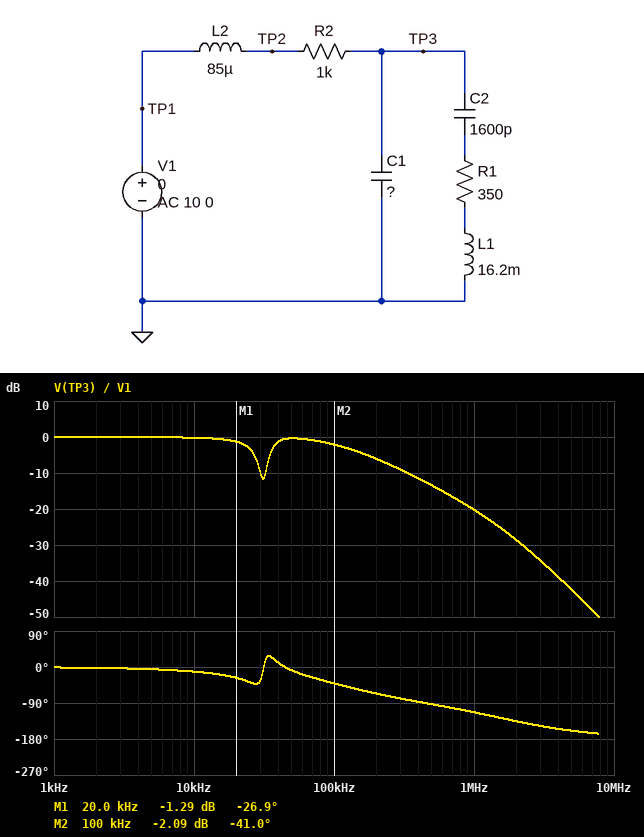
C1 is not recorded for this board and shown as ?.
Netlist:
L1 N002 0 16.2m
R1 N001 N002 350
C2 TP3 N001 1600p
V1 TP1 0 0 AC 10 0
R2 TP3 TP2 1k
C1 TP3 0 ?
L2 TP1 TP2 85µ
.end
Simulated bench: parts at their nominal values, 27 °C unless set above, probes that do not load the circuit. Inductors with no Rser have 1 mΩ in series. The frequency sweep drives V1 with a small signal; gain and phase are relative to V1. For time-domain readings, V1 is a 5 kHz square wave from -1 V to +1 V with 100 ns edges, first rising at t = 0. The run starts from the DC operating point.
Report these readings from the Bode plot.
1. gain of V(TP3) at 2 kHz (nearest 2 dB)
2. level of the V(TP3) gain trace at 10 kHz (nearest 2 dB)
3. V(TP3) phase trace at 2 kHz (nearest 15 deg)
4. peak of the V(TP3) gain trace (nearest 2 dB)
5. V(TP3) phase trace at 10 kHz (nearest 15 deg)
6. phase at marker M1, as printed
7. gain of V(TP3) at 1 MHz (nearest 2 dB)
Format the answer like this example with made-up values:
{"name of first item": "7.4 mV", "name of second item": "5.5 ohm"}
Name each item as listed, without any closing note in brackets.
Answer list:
{"gain of V(TP3) at 2 kHz": "0 dB", "level of the V(TP3) gain trace at 10 kHz": "0 dB", "V(TP3) phase trace at 2 kHz": "0 deg", "peak of the V(TP3) gain trace": "0 dB", "V(TP3) phase trace at 10 kHz": "-15 deg", "phase at marker M1, as printed": "-26.9 deg", "gain of V(TP3) at 1 MHz": "-20 dB"}
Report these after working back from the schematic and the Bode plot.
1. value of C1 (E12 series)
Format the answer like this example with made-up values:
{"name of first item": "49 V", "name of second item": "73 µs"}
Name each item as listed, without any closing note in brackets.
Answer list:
{"value of C1": "1.5 nF"}
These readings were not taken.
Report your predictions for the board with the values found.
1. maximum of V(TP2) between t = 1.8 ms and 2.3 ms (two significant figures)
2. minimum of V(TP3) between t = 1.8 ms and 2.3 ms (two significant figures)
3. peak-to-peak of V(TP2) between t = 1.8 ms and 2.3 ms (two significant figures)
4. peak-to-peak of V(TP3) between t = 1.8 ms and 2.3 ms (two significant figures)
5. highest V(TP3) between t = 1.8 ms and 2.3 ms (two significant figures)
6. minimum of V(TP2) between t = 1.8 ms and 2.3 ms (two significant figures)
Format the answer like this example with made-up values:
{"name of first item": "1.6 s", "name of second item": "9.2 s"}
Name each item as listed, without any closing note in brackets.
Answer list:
{"maximum of V(TP2) between t = 1.8 ms and 2.3 ms": "1.1 V", "minimum of V(TP3) between t = 1.8 ms and 2.3 ms": "-1.2 V", "peak-to-peak of V(TP2) between t = 1.8 ms and 2.3 ms": "2.2 V", "peak-to-peak of V(TP3) between t = 1.8 ms and 2.3 ms": "2.5 V", "highest V(TP3) between t = 1.8 ms and 2.3 ms": "1.2 V", "minimum of V(TP2) between t = 1.8 ms and 2.3 ms": "-1.1 V"}
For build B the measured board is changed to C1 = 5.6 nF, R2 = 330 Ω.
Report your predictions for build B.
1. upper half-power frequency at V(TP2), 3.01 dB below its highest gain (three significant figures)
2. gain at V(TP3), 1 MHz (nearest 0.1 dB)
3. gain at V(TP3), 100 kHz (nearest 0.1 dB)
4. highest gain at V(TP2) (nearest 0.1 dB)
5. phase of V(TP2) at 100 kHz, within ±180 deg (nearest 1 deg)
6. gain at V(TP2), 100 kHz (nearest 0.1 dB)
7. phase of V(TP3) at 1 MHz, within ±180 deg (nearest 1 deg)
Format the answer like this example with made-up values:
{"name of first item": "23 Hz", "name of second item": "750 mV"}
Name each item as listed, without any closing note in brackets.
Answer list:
{"upper half-power frequency at V(TP2), 3.01 dB below its highest gain": "605 kHz", "gain at V(TP3), 1 MHz": "-26.5 dB", "gain at V(TP3), 100 kHz": "-2.9 dB", "highest gain at V(TP2)": "0.8 dB", "phase of V(TP2) at 100 kHz, within ±180 deg": "-6 deg", "gain at V(TP2), 100 kHz": "0.7 dB", "phase of V(TP3) at 1 MHz, within ±180 deg": "-147 deg"}
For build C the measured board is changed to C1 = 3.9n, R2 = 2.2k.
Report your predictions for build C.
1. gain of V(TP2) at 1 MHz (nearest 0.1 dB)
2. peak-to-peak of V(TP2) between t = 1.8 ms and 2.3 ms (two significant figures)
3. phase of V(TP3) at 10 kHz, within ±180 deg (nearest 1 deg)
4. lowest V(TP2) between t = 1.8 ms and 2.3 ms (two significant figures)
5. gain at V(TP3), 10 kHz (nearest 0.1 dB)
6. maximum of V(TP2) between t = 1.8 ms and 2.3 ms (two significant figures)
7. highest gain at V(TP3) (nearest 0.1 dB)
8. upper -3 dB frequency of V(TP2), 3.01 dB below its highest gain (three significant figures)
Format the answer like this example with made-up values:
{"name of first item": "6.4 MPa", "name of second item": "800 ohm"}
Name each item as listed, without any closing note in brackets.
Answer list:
{"gain of V(TP2) at 1 MHz": "-0.2 dB", "peak-to-peak of V(TP2) between t = 1.8 ms and 2.3 ms": "2.0 V", "phase of V(TP3) at 10 kHz, within ±180 deg": "-38 deg", "lowest V(TP2) between t = 1.8 ms and 2.3 ms": "-1.0 V", "gain at V(TP3), 10 kHz": "-2.1 dB", "maximum of V(TP2) between t = 1.8 ms and 2.3 ms": "1.0 V", "highest gain at V(TP3)": "0 dB", "upper -3 dB frequency of V(TP2), 3.01 dB below its highest gain": "4.10 MHz"}
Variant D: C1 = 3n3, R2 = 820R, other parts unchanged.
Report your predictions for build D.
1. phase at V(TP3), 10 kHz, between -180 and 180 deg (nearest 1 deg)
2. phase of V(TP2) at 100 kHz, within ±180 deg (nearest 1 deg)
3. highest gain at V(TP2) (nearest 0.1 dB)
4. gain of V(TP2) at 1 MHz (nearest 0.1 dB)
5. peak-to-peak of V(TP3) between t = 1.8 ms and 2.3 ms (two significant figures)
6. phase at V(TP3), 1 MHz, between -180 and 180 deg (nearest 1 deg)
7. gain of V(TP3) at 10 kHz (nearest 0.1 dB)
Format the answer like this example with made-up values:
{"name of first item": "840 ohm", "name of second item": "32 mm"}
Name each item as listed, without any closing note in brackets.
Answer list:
{"phase at V(TP3), 10 kHz, between -180 and 180 deg": "-15 deg", "phase of V(TP2) at 100 kHz, within ±180 deg": "-3 deg", "highest gain at V(TP2)": "0.3 dB", "gain of V(TP2) at 1 MHz": "-1.3 dB", "peak-to-peak of V(TP3) between t = 1.8 ms and 2.3 ms": "2.4 V", "phase at V(TP3), 1 MHz, between -180 and 180 deg": "-121 deg", "gain of V(TP3) at 10 kHz": "-0.3 dB"}
